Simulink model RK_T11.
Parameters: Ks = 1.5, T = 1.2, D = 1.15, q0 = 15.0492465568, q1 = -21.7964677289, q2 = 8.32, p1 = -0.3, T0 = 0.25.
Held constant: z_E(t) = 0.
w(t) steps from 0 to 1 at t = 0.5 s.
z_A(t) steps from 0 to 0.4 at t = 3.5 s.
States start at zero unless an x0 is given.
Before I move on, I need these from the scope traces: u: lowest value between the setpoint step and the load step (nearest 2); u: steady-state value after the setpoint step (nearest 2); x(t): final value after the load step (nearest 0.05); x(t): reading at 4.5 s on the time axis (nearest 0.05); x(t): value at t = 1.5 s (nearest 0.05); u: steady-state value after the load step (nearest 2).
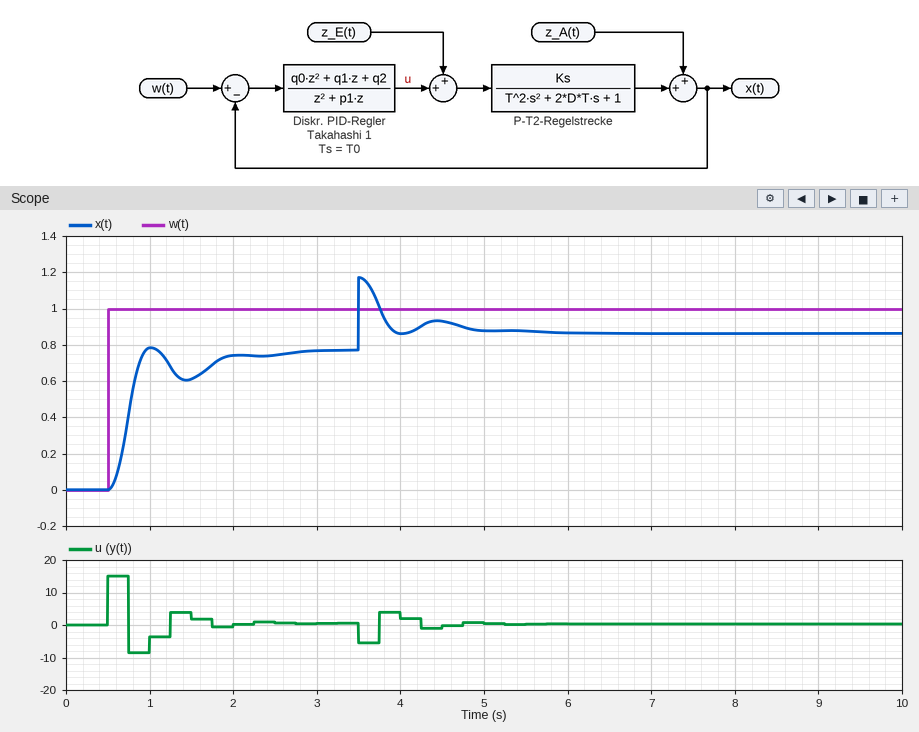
-8
0
0.85
0.95
0.60
0
